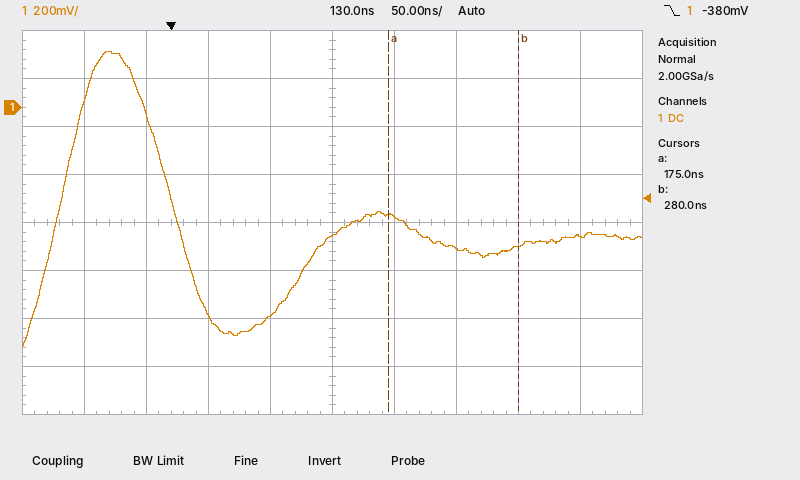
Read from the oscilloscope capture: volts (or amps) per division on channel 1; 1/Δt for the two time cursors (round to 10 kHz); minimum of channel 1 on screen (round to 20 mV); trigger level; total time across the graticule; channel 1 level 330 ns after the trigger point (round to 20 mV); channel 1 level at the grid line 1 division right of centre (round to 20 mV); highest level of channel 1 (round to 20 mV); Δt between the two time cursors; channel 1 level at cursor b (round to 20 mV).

200 mV
9.52 MHz
-1.00 V
-380 mV
500 ns
-540 mV
-460 mV
240 mV
105 ns
-580 mV
